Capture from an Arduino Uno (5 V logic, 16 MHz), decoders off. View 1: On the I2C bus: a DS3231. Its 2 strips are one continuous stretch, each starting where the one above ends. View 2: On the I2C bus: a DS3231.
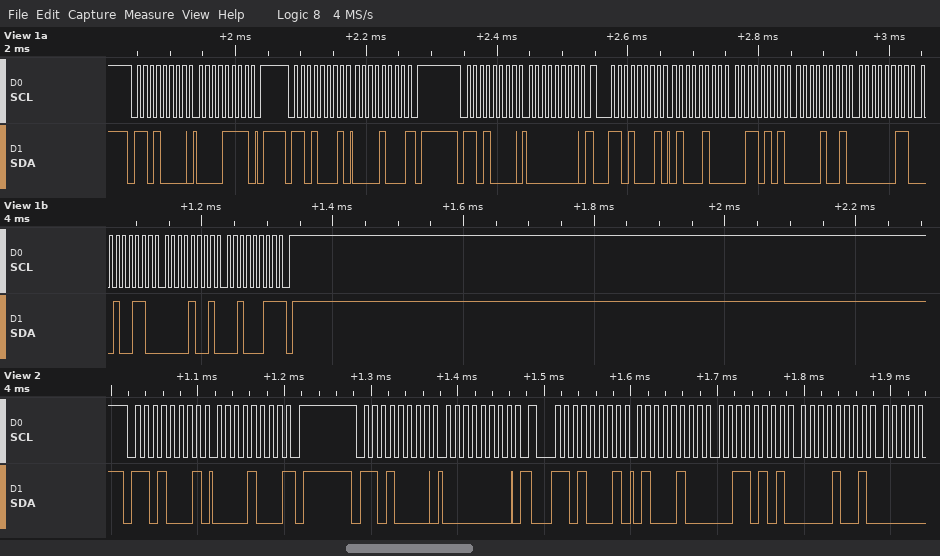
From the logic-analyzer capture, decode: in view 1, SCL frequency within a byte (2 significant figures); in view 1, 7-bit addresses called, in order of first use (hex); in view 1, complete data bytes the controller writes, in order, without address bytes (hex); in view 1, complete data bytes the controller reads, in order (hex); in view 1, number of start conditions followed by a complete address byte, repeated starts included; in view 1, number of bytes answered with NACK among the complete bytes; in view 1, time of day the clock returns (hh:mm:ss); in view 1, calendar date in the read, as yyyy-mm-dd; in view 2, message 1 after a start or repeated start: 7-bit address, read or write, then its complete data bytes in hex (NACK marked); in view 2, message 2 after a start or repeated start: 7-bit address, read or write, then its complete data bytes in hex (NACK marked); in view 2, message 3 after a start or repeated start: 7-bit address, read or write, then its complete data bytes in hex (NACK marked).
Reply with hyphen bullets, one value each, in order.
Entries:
- 100 kHz
- 0x68
- 0F 00
- 08 44 35 09 03 26 09 23
- 4
- 2
- 09:35:44
- 2023-09-26
- 0x68 read: 08 NACK
- 0x68 write: 00
- 0x68 read: 44 35 09
